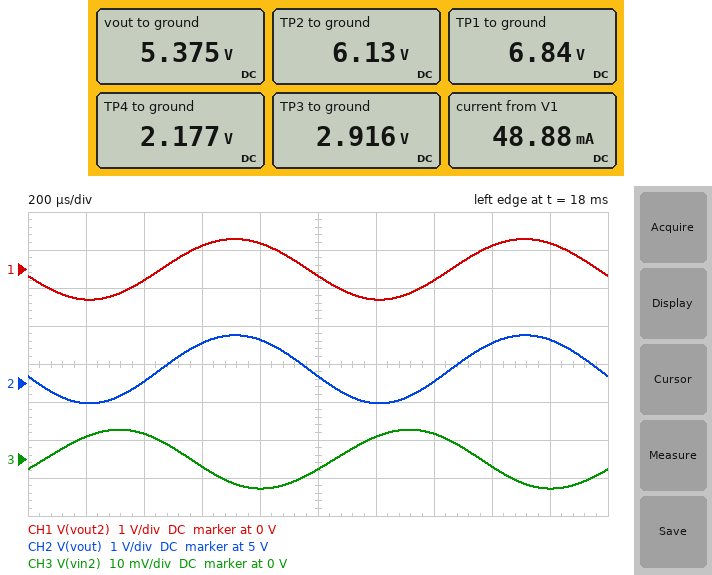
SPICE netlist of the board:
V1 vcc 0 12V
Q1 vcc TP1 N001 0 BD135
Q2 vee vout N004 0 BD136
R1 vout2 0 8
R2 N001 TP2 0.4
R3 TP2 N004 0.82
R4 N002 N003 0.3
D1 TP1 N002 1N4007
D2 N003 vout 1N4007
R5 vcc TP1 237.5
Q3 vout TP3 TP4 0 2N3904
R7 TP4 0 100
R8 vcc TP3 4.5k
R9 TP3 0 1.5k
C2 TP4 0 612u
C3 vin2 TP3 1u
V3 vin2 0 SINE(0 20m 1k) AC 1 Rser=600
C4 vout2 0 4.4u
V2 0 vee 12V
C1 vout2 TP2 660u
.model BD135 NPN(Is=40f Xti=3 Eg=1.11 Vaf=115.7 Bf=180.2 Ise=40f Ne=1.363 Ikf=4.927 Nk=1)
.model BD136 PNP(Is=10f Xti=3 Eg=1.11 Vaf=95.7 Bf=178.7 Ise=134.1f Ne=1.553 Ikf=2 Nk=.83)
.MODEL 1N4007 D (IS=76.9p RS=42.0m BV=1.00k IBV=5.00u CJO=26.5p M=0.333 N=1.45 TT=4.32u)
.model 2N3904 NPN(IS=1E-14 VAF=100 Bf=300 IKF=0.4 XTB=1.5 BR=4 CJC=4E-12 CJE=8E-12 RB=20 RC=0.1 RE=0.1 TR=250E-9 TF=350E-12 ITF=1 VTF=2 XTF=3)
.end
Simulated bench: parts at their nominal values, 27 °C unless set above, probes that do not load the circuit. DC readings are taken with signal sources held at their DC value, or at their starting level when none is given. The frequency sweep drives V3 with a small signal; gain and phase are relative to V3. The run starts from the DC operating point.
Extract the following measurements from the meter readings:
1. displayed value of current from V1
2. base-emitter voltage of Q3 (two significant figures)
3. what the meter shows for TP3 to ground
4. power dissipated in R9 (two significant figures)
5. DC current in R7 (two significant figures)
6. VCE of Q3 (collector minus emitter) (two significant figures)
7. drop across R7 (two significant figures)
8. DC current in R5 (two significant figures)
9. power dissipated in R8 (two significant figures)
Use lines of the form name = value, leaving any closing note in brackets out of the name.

displayed value of current from V1 = 48.88 mA
base-emitter voltage of Q3 = 740 mV
what the meter shows for TP3 to ground = 2.916 V
power dissipated in R9 = 5.7 mW
DC current in R7 = 22 mA
VCE of Q3 (collector minus emitter) = 3.2 V
drop across R7 = 2.2 V
DC current in R5 = 22 mA
power dissipated in R8 = 18 mW
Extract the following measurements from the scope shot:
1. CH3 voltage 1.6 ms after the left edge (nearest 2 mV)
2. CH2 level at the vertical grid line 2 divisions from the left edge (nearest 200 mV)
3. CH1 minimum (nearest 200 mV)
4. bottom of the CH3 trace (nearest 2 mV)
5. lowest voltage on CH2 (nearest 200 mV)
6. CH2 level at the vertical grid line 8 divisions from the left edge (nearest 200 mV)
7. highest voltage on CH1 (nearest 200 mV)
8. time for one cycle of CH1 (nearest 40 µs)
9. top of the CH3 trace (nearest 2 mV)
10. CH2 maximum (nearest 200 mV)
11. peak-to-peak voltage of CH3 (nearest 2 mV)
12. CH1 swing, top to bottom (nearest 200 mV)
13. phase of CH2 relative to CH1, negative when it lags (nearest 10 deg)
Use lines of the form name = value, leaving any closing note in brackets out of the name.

CH3 voltage 1.6 ms after the left edge = -2 mV
CH2 level at the vertical grid line 2 divisions from the left edge = 5.0 V
CH1 minimum = -800 mV
bottom of the CH3 trace = -8 mV
lowest voltage on CH2 = 4.4 V
CH2 level at the vertical grid line 8 divisions from the left edge = 6.0 V
highest voltage on CH1 = 800 mV
time for one cycle of CH1 = 1.00 ms
top of the CH3 trace = 8 mV
CH2 maximum = 6.2 V
peak-to-peak voltage of CH3 = 16 mV
CH1 swing, top to bottom = 1.6 V
phase of CH2 relative to CH1, negative when it lags = 0 deg
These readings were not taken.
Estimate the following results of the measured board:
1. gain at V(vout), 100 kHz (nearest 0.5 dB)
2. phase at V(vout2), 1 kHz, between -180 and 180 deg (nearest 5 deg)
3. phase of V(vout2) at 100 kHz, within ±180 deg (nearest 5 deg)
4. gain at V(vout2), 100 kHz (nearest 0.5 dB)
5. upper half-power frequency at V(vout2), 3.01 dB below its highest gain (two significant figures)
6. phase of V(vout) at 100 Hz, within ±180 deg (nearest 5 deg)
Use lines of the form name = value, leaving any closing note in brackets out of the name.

gain at V(vout), 100 kHz = 27.0 dB
phase at V(vout2), 1 kHz, between -180 and 180 deg = -165 deg
phase of V(vout2) at 100 kHz, within ±180 deg = 100 deg
gain at V(vout2), 100 kHz = 19.0 dB
upper half-power frequency at V(vout2), 3.01 dB below its highest gain = 22 kHz
phase of V(vout) at 100 Hz, within ±180 deg = -95 deg
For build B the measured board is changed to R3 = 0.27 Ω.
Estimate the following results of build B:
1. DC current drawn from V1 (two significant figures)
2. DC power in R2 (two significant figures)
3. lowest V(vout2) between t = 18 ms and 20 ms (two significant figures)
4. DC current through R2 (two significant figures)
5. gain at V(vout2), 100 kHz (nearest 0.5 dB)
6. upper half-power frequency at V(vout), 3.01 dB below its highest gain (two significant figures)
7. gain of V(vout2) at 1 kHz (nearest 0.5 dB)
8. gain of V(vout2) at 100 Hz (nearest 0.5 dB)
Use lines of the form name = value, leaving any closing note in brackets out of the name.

DC current drawn from V1 = 54 mA
DC power in R2 = 380 µW
lowest V(vout2) between t = 18 ms and 20 ms = -840 mV
DC current through R2 = 31 mA
gain at V(vout2), 100 kHz = 20.0 dB
upper half-power frequency at V(vout), 3.01 dB below its highest gain = 28 kHz
gain of V(vout2) at 1 kHz = 32.5 dB
gain of V(vout2) at 100 Hz = 23.5 dB
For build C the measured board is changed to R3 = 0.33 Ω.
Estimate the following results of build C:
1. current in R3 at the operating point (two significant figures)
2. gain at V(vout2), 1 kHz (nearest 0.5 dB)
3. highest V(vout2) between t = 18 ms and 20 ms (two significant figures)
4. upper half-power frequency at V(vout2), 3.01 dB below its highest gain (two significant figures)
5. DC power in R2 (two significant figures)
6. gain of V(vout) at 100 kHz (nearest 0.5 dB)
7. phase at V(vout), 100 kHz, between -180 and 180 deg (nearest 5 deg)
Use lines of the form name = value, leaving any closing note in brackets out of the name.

current in R3 at the operating point = 30 mA
gain at V(vout2), 1 kHz = 32.5 dB
highest V(vout2) between t = 18 ms and 20 ms = 800 mV
upper half-power frequency at V(vout2), 3.01 dB below its highest gain = 24 kHz
DC power in R2 = 360 µW
gain of V(vout) at 100 kHz = 26.0 dB
phase at V(vout), 100 kHz, between -180 and 180 deg = 160 deg
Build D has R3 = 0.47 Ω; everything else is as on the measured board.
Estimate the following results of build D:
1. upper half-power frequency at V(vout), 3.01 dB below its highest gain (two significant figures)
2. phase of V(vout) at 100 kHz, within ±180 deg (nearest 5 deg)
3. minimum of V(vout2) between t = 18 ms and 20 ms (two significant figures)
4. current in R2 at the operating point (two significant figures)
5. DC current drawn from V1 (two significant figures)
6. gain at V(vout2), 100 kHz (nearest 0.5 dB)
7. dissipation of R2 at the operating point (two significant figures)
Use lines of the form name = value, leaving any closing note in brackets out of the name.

upper half-power frequency at V(vout), 3.01 dB below its highest gain = 28 kHz
phase of V(vout) at 100 kHz, within ±180 deg = 160 deg
minimum of V(vout2) between t = 18 ms and 20 ms = -830 mV
current in R2 at the operating point = 28 mA
DC current drawn from V1 = 52 mA
gain at V(vout2), 100 kHz = 19.5 dB
dissipation of R2 at the operating point = 320 µW
